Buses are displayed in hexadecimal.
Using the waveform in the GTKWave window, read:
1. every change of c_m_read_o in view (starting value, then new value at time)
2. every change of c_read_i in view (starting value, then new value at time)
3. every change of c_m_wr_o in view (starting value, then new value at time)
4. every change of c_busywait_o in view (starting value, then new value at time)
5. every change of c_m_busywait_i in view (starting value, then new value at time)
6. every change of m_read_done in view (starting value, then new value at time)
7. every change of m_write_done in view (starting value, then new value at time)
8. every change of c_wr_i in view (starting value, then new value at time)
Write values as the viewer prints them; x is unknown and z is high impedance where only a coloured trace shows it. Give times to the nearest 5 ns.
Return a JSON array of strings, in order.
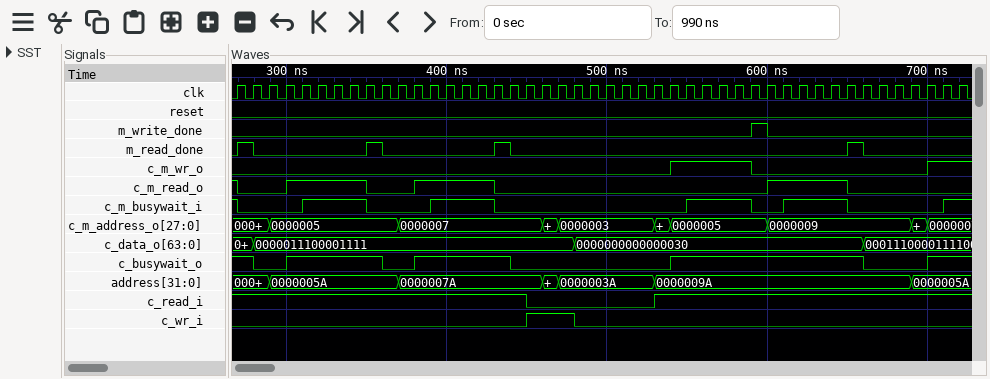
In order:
["1, 0 at 270 ns, 1 at 300 ns, 0 at 350 ns, 1 at 380 ns, 0 at 430 ns, 1 at 600 ns, 0 at 650 ns", "1, 0 at 450 ns, 1 at 530 ns", "0, 1 at 540 ns, 0 at 590 ns, 1 at 700 ns", "1, 0 at 280 ns, 1 at 300 ns, 0 at 360 ns, 1 at 380 ns, 0 at 440 ns, 1 at 540 ns, 0 at 660 ns, 1 at 700 ns", "1, 0 at 270 ns, 1 at 310 ns, 0 at 350 ns, 1 at 390 ns, 0 at 430 ns, 1 at 550 ns, 0 at 590 ns, 1 at 610 ns, 0 at 650 ns, 1 at 710 ns", "0, 1 at 270 ns, 0 at 280 ns, 1 at 350 ns, 0 at 360 ns, 1 at 430 ns, 0 at 440 ns, 1 at 650 ns, 0 at 660 ns", "0, 1 at 590 ns, 0 at 600 ns", "0, 1 at 450 ns, 0 at 480 ns"]
